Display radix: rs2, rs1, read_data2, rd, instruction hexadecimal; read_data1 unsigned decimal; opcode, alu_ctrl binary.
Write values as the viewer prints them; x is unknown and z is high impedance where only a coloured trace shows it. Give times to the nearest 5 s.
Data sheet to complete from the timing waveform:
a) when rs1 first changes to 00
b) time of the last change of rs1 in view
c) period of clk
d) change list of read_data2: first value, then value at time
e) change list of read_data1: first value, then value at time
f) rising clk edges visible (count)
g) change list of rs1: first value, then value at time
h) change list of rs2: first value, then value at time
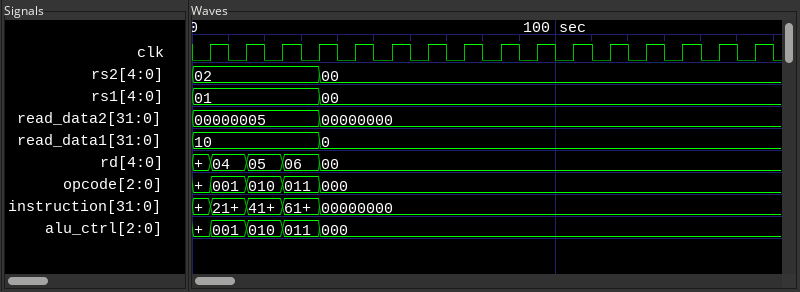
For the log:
35 s
35 s
10 s
00000005, 00000000 at 35 s
10, 0 at 35 s
16
01, 00 at 35 s
02, 00 at 35 s
